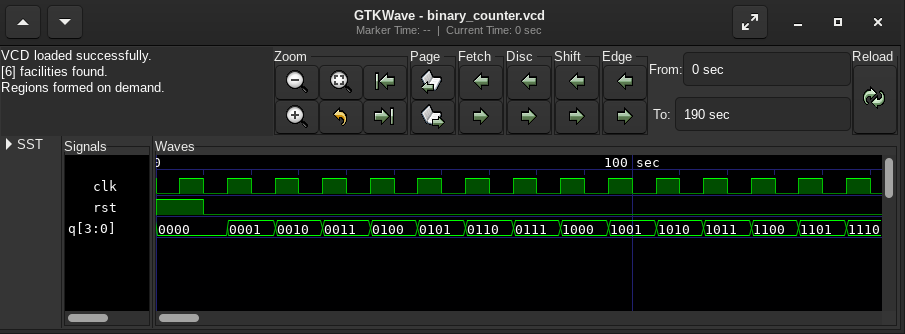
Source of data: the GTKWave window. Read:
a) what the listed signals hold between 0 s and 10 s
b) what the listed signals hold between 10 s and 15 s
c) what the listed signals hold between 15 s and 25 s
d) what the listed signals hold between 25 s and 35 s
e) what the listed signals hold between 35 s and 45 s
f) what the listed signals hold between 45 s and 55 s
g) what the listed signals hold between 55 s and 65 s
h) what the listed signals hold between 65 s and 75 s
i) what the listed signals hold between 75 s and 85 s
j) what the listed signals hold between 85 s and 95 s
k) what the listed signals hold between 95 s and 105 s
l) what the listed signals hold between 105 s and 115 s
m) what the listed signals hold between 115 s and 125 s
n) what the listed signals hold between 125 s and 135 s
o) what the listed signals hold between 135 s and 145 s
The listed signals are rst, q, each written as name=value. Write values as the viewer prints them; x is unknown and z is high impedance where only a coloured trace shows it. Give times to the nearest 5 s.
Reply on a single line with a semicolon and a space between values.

rst=1, q=0000; rst=0, q=0000; rst=0, q=0001; rst=0, q=0010; rst=0, q=0011; rst=0, q=0100; rst=0, q=0101; rst=0, q=0110; rst=0, q=0111; rst=0, q=1000; rst=0, q=1001; rst=0, q=1010; rst=0, q=1011; rst=0, q=1100; rst=0, q=1101
